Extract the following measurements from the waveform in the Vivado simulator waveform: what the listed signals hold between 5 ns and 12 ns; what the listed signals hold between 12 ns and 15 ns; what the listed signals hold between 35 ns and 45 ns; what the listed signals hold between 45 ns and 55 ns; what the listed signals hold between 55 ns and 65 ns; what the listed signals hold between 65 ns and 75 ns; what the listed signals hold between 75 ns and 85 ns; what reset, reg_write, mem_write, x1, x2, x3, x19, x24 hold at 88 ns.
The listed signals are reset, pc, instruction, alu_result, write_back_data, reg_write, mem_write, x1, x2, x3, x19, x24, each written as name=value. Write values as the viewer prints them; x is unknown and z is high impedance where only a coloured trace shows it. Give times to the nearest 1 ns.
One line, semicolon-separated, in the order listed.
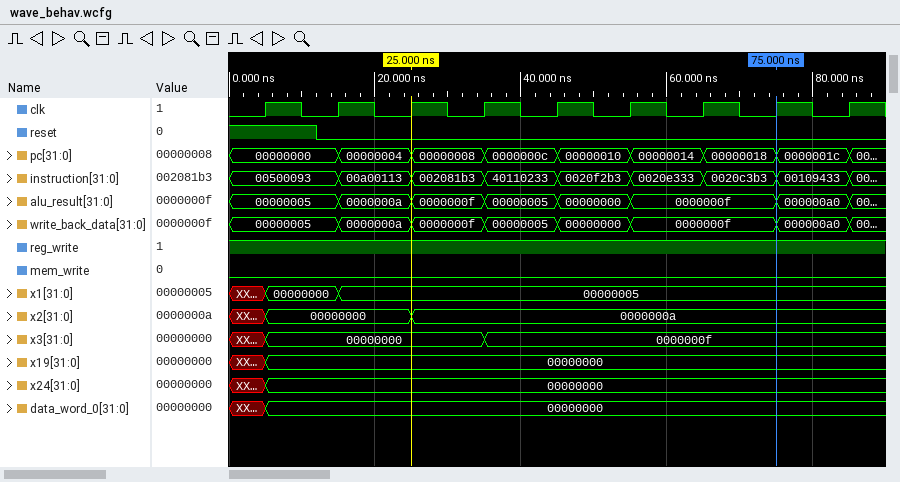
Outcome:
reset=1, pc=00000000, instruction=00500093, alu_result=00000005, write_back_data=00000005, reg_write=1, mem_write=0, x1=00000000, x2=00000000, x3=00000000, x19=00000000, x24=00000000; reset=0, pc=00000000, instruction=00500093, alu_result=00000005, write_back_data=00000005, reg_write=1, mem_write=0, x1=00000000, x2=00000000, x3=00000000, x19=00000000, x24=00000000; reset=0, pc=0000000c, instruction=40110233, alu_result=00000005, write_back_data=00000005, reg_write=1, mem_write=0, x1=00000005, x2=0000000a, x3=0000000f, x19=00000000, x24=00000000; reset=0, pc=00000010, instruction=0020f2b3, alu_result=00000000, write_back_data=00000000, reg_write=1, mem_write=0, x1=00000005, x2=0000000a, x3=0000000f, x19=00000000, x24=00000000; reset=0, pc=00000014, instruction=0020e333, alu_result=0000000f, write_back_data=0000000f, reg_write=1, mem_write=0, x1=00000005, x2=0000000a, x3=0000000f, x19=00000000, x24=00000000; reset=0, pc=00000018, instruction=0020c3b3, alu_result=0000000f, write_back_data=0000000f, reg_write=1, mem_write=0, x1=00000005, x2=0000000a, x3=0000000f, x19=00000000, x24=00000000; reset=0, pc=0000001c, instruction=00109433, alu_result=000000a0, write_back_data=000000a0, reg_write=1, mem_write=0, x1=00000005, x2=0000000a, x3=0000000f, x19=00000000, x24=00000000; reset=0, reg_write=1, mem_write=0, x1=00000005, x2=0000000a, x3=0000000f, x19=00000000, x24=00000000
